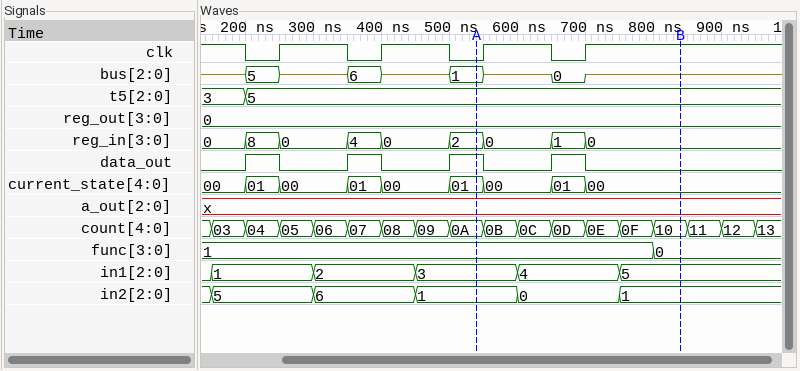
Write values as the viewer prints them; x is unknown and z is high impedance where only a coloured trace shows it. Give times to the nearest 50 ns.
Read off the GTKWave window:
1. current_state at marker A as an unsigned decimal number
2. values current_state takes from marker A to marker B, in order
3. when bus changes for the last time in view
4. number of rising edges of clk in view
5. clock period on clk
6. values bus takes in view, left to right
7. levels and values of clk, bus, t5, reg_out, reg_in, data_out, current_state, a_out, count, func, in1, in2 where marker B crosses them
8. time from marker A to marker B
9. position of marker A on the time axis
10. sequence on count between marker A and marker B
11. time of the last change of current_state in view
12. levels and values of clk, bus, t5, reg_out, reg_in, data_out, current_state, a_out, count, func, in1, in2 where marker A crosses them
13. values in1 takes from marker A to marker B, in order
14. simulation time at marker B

1
01, 00, 01, 00
700 ns
4
150 ns
z, 5, z, 6, z, 1, z, 0, z
clk=1, bus=z, t5=5, reg_out=0, reg_in=0, data_out=0, current_state=00, a_out=x, count=10, func=0, in1=5, in2=1
300 ns
550 ns
0A, 0B, 0C, 0D, 0E, 0F, 10
700 ns
clk=0, bus=1, t5=5, reg_out=0, reg_in=2, data_out=1, current_state=01, a_out=x, count=0A, func=1, in1=3, in2=1
3, 4, 5
850 ns
